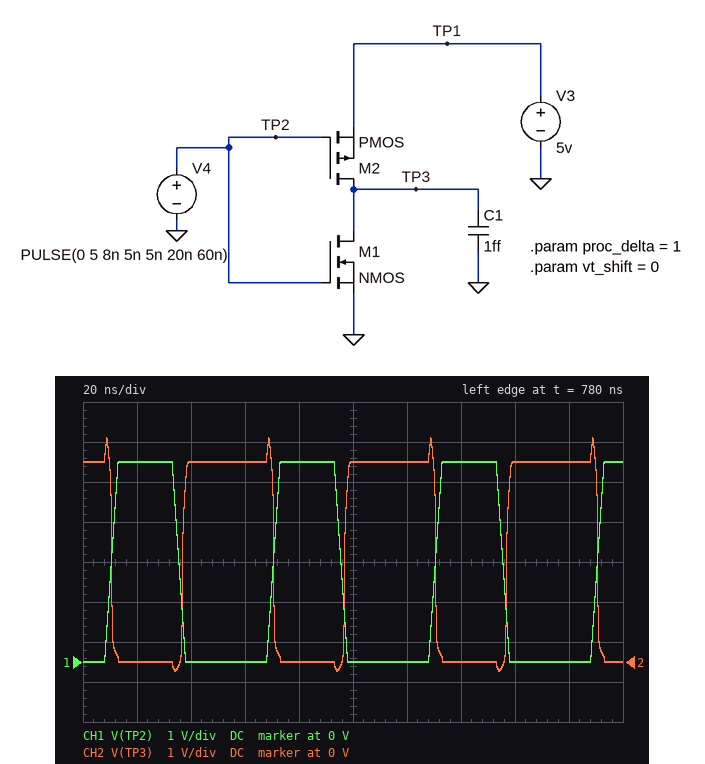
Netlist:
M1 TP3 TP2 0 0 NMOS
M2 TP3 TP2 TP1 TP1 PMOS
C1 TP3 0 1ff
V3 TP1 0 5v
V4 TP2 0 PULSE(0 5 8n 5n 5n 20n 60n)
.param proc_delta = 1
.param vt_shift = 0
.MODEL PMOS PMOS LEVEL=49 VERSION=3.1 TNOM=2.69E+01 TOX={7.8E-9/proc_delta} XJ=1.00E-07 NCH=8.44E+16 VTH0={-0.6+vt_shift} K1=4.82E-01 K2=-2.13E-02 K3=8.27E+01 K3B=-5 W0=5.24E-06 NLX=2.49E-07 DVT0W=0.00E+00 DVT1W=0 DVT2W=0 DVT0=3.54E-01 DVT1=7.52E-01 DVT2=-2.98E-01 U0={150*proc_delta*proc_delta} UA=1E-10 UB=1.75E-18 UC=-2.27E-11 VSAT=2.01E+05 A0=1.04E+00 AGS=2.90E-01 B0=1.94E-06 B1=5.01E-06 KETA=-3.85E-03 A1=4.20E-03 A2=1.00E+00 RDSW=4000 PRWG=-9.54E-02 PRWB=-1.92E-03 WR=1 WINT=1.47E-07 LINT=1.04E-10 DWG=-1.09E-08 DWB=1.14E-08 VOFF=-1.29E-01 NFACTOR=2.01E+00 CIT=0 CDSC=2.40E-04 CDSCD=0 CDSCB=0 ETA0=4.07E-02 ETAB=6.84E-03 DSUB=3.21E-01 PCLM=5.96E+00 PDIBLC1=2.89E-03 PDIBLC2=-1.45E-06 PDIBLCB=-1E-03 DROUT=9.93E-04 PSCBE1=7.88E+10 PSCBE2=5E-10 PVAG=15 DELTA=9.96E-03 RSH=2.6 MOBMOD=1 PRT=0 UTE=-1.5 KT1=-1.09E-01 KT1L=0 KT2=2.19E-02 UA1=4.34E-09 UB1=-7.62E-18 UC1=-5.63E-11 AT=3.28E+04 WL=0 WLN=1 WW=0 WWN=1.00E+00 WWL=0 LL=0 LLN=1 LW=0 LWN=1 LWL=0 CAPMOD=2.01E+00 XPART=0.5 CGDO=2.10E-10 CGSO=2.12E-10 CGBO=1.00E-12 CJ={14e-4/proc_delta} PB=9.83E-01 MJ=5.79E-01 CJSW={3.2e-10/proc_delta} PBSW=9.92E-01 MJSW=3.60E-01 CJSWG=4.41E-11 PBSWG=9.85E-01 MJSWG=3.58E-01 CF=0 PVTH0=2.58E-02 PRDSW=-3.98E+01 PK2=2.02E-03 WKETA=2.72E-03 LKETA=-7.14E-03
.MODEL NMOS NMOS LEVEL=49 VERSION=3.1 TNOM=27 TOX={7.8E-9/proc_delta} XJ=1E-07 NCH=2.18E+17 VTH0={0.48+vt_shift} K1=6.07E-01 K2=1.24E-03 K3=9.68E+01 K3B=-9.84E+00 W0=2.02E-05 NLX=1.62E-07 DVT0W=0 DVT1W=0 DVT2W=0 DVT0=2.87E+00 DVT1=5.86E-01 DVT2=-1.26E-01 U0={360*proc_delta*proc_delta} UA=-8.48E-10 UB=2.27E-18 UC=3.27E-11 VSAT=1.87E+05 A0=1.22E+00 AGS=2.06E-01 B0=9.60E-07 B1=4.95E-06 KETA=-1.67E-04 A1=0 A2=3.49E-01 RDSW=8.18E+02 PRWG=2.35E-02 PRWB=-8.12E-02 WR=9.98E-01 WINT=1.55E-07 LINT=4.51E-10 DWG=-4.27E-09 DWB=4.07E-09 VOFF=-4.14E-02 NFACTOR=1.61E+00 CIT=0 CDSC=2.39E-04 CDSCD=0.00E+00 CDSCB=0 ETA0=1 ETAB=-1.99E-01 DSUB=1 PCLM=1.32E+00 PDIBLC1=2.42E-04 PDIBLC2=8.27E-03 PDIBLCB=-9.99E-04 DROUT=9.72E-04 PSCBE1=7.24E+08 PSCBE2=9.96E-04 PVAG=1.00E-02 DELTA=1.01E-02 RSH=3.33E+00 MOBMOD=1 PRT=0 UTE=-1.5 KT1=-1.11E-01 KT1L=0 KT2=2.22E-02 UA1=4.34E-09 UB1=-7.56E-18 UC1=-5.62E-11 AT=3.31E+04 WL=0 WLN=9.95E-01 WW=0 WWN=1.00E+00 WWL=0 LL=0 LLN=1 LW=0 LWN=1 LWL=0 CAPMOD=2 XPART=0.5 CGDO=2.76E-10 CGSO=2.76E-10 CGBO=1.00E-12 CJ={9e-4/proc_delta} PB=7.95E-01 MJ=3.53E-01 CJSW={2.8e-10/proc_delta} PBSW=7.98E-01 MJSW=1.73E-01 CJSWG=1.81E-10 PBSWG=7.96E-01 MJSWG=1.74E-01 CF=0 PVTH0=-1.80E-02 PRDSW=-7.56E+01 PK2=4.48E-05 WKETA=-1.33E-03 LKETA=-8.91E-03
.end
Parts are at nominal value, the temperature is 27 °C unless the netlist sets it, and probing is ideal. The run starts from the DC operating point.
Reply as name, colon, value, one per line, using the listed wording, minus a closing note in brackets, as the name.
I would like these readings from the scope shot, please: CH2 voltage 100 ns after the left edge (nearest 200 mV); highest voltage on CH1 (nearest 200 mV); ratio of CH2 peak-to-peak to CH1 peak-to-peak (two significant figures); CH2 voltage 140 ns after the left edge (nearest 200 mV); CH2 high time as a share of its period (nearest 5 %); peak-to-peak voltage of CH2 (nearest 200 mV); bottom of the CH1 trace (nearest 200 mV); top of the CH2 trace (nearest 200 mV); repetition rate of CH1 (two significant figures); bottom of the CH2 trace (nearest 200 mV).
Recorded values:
CH2 voltage 100 ns after the left edge: 5.0 V
highest voltage on CH1: 5.0 V
ratio of CH2 peak-to-peak to CH1 peak-to-peak: 1.2
CH2 voltage 140 ns after the left edge: 0 V
CH2 high time as a share of its period: 55 %
peak-to-peak voltage of CH2: 5.8 V
bottom of the CH1 trace: 0 V
top of the CH2 trace: 5.6 V
repetition rate of CH1: 17 MHz
bottom of the CH2 trace: -200 mV
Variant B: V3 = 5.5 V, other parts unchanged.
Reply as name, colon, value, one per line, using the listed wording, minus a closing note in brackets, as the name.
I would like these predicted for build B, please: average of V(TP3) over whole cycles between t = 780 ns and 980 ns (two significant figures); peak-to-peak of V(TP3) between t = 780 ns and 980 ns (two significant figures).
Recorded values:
average of V(TP3) over whole cycles between t = 780 ns and 980 ns: 3.1 V
peak-to-peak of V(TP3) between t = 780 ns and 980 ns: 6.3 V
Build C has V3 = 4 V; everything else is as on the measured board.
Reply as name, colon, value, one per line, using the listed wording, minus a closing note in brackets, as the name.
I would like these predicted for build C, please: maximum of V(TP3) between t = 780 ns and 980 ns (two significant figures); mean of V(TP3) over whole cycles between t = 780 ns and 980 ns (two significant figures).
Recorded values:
maximum of V(TP3) between t = 780 ns and 980 ns: 4.7 V
mean of V(TP3) over whole cycles between t = 780 ns and 980 ns: 2.2 V
